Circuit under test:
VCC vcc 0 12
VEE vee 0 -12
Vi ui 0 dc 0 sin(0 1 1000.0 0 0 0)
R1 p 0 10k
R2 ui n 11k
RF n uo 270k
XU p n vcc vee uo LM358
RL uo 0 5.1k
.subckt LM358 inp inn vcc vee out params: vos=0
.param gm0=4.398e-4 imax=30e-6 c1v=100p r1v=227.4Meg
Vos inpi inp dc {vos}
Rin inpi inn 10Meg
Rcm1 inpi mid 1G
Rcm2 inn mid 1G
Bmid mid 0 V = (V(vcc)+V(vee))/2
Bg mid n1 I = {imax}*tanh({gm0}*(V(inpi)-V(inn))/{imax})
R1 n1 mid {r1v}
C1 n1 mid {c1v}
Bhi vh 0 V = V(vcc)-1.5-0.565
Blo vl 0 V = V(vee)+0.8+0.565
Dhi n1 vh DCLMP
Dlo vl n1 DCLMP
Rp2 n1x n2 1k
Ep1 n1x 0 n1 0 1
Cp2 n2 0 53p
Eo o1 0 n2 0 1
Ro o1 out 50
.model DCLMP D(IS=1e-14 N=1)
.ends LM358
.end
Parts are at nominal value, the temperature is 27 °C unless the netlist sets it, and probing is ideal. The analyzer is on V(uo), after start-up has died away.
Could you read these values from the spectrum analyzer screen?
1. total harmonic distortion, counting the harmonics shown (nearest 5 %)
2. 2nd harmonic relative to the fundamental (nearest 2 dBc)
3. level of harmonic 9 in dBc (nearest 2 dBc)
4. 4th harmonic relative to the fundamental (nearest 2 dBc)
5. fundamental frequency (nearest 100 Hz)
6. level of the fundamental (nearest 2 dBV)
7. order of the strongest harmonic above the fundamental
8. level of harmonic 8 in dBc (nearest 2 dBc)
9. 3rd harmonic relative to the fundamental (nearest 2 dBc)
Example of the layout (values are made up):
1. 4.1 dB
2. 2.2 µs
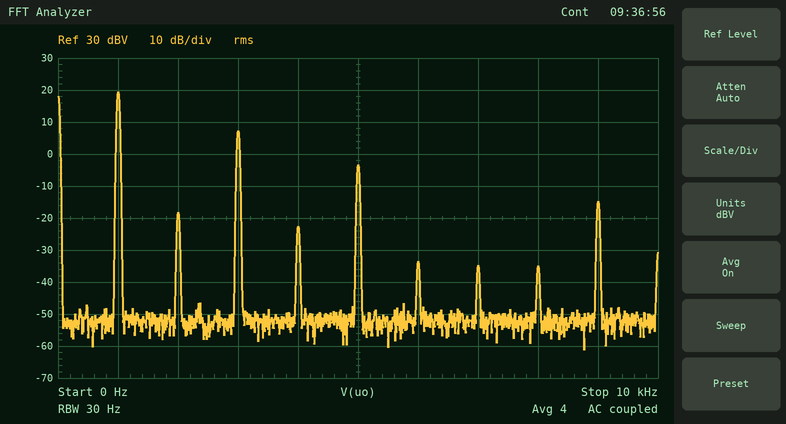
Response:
1. 25 %
2. -38 dBc
3. -34 dBc
4. -42 dBc
5. 1.0 kHz
6. 20 dBV
7. 3
8. -54 dBc
9. -12 dBc
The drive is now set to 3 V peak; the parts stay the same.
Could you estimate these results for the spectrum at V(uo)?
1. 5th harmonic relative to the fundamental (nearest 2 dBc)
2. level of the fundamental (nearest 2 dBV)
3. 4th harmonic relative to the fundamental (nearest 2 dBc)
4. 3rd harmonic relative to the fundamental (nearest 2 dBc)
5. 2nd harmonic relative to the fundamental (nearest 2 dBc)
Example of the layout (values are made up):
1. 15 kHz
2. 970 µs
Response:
1. -16 dBc
2. 20 dBV
3. -48 dBc
4. -10 dBc
5. -46 dBc
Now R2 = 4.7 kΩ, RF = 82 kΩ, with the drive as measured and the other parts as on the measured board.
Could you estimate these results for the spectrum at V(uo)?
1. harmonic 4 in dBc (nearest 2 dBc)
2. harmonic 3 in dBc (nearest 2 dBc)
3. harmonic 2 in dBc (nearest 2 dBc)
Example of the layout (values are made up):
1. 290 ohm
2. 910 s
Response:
1. -48 dBc
2. -16 dBc
3. -36 dBc
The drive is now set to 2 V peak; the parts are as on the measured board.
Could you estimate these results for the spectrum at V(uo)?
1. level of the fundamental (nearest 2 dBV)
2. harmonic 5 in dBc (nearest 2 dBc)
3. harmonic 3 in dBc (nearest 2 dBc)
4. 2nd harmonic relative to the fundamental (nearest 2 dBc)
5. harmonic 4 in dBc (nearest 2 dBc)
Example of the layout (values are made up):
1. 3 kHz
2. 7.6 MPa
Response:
1. 20 dBV
2. -16 dBc
3. -10 dBc
4. -44 dBc
5. -44 dBc
